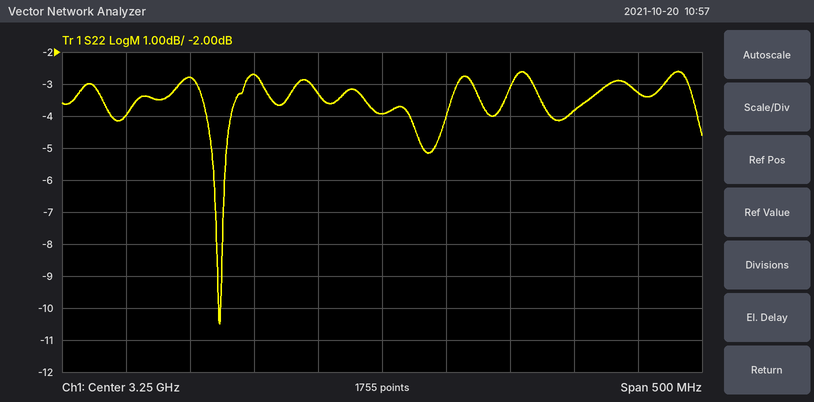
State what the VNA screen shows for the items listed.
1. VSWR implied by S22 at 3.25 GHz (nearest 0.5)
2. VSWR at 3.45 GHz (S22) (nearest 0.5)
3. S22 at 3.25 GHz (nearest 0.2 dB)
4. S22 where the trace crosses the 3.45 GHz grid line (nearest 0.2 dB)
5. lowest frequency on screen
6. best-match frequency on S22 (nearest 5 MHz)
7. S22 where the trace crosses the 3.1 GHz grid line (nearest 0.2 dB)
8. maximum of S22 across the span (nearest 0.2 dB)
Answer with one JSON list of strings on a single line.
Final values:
["4.5", "5.5", "-4.0 dB", "-3.2 dB", "3 GHz", "3.125 GHz", "-2.8 dB", "-2.6 dB"]
